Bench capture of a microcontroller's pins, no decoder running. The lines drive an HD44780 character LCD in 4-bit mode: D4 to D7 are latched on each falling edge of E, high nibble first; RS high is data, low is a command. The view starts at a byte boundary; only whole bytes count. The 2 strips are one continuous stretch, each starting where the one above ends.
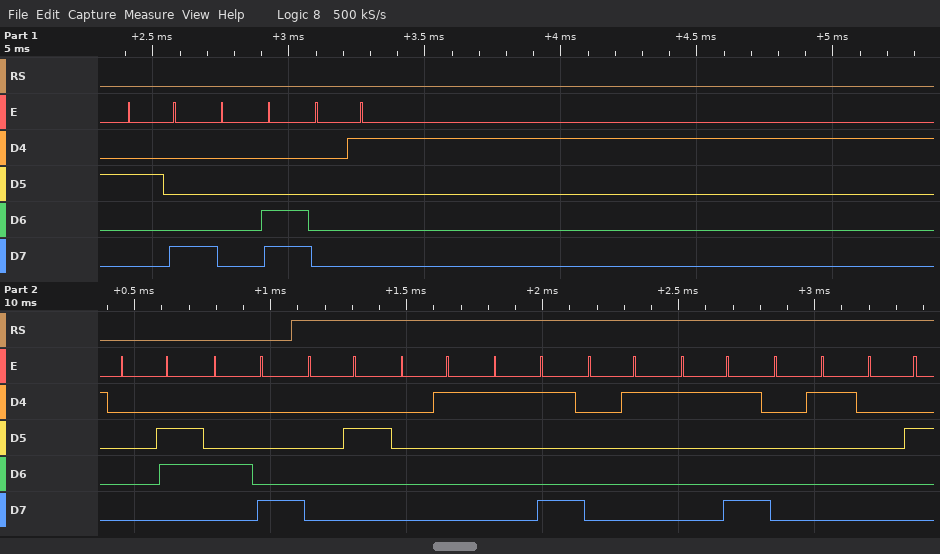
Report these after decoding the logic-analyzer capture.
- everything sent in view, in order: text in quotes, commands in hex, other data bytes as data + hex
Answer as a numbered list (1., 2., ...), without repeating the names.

1. 0x28 0x0C 0x01 0x06 0x48 data 02 01 19 01 19 01 02
